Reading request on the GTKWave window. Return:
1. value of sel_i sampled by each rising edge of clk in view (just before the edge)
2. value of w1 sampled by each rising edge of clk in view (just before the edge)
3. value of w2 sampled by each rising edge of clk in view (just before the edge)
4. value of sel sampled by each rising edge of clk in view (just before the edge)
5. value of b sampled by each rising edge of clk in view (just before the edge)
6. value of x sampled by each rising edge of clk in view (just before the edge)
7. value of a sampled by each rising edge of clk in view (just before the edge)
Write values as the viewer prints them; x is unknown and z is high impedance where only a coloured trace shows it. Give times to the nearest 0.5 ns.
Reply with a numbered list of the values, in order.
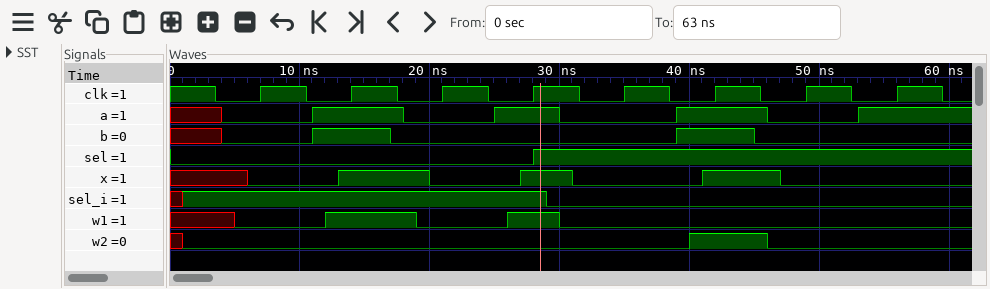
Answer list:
1. 1 1 1 1 0 0 0 0
2. 0 1 0 1 0 0 0 0
3. 0 0 0 0 0 1 0 0
4. 0 0 0 0 1 1 1 1
5. 0 1 0 0 0 1 0 0
6. 0 1 0 1 0 1 0 0
7. 0 1 0 1 0 1 0 1
